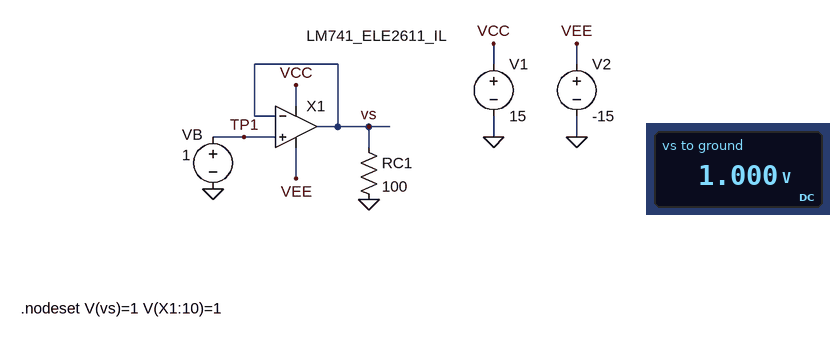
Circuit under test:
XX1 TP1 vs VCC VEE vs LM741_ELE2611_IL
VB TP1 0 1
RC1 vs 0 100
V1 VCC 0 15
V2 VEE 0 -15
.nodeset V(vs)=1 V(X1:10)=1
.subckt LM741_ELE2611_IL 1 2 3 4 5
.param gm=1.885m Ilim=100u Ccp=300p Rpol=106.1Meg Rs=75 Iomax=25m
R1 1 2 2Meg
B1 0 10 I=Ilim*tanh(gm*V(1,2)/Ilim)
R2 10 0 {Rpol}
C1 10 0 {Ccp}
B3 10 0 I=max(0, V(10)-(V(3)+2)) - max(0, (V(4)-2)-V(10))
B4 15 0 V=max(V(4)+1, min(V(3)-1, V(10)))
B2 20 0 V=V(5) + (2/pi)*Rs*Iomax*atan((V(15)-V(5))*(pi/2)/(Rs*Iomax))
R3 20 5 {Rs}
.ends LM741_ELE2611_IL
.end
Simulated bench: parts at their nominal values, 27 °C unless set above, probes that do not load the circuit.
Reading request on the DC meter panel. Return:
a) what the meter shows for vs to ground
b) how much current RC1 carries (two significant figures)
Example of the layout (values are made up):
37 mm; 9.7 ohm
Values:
1.000 V; 10 mA
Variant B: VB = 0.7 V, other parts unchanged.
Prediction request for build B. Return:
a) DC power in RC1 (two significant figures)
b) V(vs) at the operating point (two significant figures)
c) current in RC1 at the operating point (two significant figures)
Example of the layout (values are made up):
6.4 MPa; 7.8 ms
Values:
4.9 mW; 700 mV; 7.0 mA
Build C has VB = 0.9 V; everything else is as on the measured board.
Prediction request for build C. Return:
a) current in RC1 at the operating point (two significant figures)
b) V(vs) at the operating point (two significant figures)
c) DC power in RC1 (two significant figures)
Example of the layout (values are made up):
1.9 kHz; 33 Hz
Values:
9.0 mA; 900 mV; 8.1 mW
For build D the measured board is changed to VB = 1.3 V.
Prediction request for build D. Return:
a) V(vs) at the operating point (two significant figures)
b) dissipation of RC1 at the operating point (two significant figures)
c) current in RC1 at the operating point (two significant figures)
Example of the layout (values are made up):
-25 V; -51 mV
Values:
1.3 V; 17 mW; 13 mA
